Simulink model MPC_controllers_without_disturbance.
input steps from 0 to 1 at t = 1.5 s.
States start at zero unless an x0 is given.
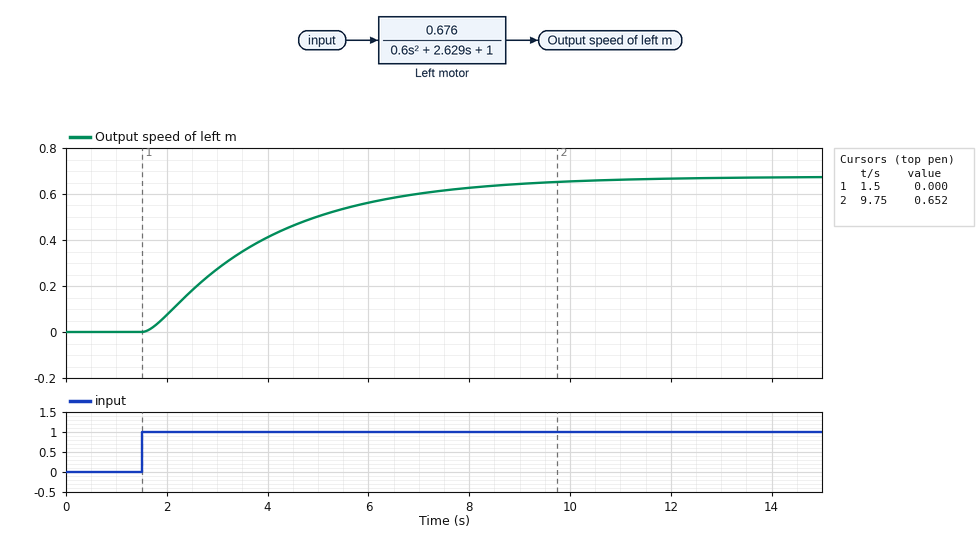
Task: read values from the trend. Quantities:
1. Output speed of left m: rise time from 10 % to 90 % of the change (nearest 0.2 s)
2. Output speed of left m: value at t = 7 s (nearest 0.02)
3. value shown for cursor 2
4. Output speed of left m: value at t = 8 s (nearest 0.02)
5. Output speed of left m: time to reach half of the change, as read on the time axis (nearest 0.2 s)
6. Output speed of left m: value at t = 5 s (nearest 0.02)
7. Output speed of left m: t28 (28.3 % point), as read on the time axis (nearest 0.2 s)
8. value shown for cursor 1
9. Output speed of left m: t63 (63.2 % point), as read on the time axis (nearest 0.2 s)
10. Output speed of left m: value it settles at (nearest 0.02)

5.2 s
0.60
0.652
0.62
3.4 s
0.50
2.6 s
0.000
4.2 s
0.68
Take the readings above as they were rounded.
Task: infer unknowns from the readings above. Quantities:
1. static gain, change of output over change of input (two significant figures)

0.68
